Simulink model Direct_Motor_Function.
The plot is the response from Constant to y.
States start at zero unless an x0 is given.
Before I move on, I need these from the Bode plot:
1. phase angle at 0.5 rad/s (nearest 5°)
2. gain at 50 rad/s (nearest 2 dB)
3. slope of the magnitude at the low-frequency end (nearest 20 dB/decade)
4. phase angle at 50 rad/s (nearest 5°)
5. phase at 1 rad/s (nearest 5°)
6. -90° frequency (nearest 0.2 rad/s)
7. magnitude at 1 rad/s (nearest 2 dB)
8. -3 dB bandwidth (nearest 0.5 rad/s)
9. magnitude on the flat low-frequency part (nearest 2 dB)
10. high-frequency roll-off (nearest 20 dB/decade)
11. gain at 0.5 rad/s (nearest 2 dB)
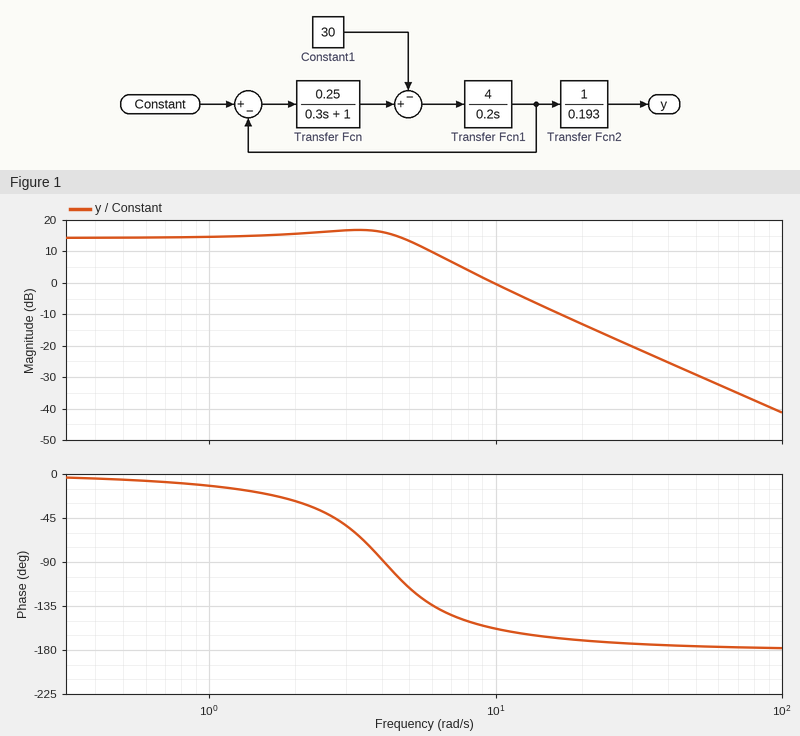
-5°
-30 dB
0 dB/decade
-175°
-10°
4.0 rad/s
14 dB
5.5 rad/s
14 dB
-40 dB/decade
14 dB
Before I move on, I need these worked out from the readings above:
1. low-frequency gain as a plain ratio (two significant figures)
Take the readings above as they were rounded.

5.0
